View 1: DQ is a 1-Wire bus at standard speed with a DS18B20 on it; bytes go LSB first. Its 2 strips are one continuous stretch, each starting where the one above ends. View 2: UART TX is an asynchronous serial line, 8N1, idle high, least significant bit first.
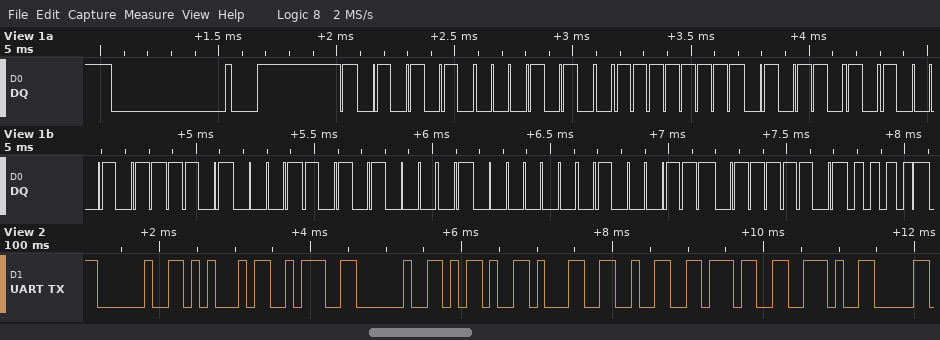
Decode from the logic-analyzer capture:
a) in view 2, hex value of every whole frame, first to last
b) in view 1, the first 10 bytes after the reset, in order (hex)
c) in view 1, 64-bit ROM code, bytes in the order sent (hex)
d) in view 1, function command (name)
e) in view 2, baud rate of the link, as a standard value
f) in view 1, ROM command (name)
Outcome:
20 45 3A 20 2D 31 32 37 2E
55 28 FF 5A D1 8B 15 02 E2 BE
28 FF 5A D1 8B 15 02 E2
Read Scratchpad
9600 baud
Match ROM
